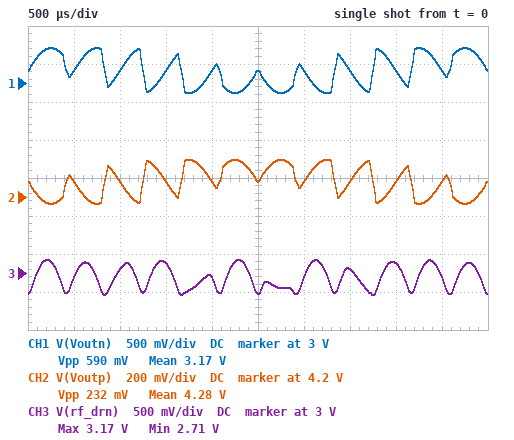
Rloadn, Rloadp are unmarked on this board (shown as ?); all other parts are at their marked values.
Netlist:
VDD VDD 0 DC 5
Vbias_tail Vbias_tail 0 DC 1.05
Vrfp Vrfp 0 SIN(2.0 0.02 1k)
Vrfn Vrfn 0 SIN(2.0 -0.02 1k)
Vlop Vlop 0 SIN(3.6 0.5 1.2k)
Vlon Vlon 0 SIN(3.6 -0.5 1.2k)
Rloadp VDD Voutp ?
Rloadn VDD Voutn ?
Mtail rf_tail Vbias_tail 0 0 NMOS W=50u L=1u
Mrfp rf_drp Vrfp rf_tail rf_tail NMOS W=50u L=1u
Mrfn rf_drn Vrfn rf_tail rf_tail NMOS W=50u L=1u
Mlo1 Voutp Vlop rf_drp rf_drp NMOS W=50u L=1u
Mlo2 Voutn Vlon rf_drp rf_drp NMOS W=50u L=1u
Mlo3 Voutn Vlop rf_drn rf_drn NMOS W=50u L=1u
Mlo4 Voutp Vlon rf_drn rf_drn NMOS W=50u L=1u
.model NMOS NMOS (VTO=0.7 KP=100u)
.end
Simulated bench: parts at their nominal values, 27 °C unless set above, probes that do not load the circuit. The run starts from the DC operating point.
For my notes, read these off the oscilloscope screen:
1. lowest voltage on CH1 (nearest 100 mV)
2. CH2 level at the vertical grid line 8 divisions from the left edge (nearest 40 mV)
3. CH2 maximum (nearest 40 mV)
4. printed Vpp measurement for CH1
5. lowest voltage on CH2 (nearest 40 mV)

2.9 V
4.28 V
4.40 V
590 mV
4.16 V
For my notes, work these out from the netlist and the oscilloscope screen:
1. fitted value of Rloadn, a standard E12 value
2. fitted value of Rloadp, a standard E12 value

12 kΩ
4.7 kΩ
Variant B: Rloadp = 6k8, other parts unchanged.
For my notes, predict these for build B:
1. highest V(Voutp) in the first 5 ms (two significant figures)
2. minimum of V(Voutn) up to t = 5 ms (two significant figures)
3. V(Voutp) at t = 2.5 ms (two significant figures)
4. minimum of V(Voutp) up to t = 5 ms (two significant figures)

4.1 V
2.9 V
4.0 V
3.8 V
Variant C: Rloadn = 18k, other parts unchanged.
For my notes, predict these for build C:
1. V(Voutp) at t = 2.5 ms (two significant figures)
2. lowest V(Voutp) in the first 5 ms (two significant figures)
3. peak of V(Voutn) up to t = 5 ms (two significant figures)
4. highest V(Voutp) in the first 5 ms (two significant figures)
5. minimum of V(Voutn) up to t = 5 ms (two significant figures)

4.1 V
4.1 V
2.8 V
4.2 V
2.5 V
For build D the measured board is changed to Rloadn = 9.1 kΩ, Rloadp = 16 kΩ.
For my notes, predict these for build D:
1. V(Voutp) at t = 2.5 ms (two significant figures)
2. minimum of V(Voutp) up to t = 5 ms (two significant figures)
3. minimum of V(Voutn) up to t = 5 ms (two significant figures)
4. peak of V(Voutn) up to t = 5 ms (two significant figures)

2.8 V
2.5 V
3.4 V
3.6 V
